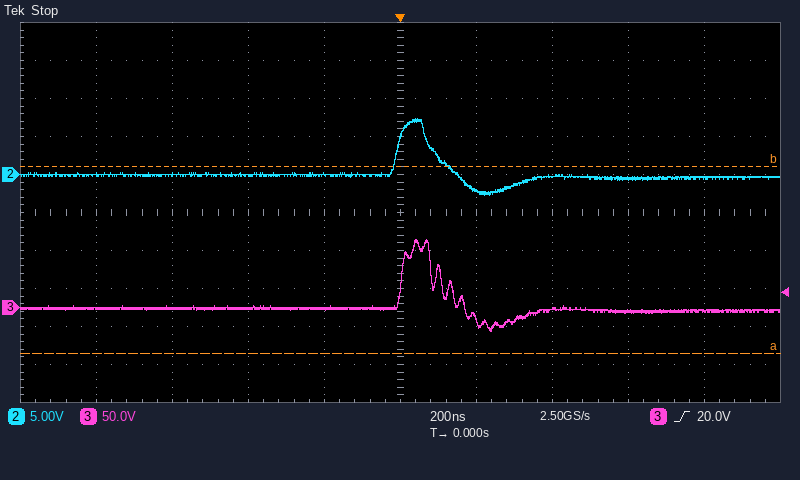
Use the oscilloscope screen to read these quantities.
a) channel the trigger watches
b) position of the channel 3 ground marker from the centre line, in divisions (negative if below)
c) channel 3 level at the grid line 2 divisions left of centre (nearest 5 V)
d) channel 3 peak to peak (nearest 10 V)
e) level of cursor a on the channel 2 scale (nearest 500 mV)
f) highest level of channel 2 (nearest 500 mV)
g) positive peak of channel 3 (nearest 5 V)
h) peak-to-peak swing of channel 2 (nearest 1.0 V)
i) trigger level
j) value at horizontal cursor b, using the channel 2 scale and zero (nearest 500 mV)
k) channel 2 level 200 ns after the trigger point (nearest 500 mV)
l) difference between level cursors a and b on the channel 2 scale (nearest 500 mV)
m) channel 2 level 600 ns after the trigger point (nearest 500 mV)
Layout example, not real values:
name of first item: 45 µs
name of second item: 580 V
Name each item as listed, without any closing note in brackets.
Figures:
channel the trigger watches: channel 3
position of the channel 3 ground marker from the centre line, in divisions: -2.5 div
channel 3 level at the grid line 2 divisions left of centre: 0 V
channel 3 peak to peak: 120 V
level of cursor a on the channel 2 scale: -23.5 V
highest level of channel 2: 7.5 V
positive peak of channel 3: 90 V
peak-to-peak swing of channel 2: 10.0 V
trigger level: 20.0 V
value at horizontal cursor b, using the channel 2 scale and zero: 1.0 V
channel 2 level 200 ns after the trigger point: -2.0 V
difference between level cursors a and b on the channel 2 scale: 24.5 V
channel 2 level 600 ns after the trigger point: -500 mV
